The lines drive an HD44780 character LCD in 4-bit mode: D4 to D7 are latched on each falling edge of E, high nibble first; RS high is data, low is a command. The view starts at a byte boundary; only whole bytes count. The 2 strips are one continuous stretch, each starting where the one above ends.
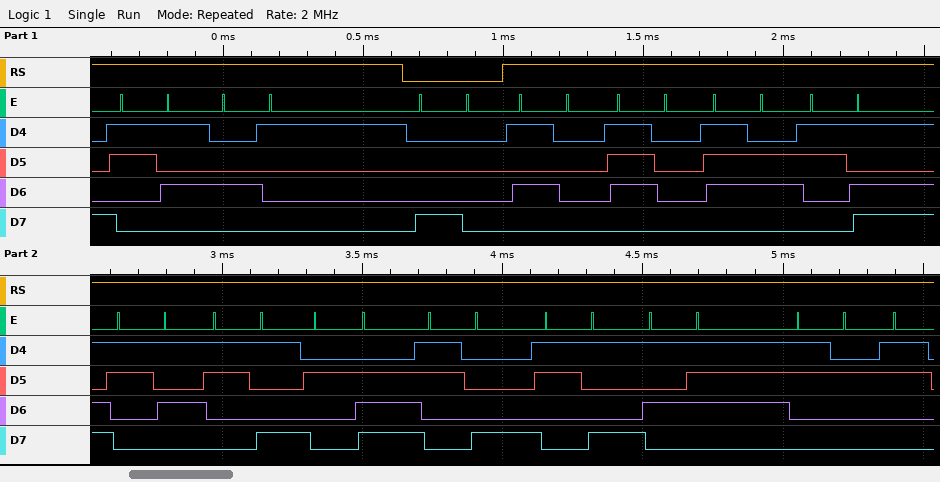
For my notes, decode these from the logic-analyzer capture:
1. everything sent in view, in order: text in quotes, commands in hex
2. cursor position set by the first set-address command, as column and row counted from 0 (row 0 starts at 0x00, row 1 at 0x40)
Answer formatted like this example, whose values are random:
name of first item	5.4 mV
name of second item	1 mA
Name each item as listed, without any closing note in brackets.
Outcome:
everything sent in view, in order: text in quotes, commands in hex	"5A" 0x80 "Ppv=59.89W2"
cursor position set by the first set-address command, as column and row counted from 0	column 0, row 0
